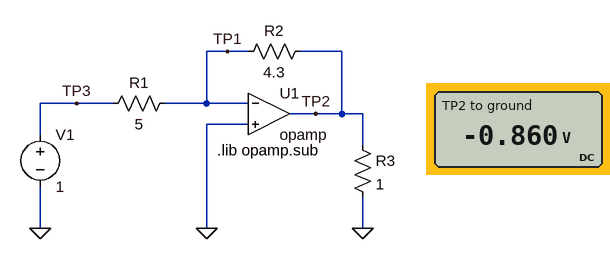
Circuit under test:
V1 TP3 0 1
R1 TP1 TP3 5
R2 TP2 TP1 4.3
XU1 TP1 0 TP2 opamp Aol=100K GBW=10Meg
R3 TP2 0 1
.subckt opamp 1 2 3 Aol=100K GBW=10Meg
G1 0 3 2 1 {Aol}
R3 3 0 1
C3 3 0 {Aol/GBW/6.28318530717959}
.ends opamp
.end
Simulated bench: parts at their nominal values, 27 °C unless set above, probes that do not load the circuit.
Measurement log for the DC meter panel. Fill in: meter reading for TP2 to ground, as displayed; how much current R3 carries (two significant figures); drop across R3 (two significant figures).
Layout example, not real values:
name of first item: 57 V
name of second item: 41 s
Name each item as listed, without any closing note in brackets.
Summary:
meter reading for TP2 to ground, as displayed: -0.860 V
how much current R3 carries: 860 mA
drop across R3: 860 mV
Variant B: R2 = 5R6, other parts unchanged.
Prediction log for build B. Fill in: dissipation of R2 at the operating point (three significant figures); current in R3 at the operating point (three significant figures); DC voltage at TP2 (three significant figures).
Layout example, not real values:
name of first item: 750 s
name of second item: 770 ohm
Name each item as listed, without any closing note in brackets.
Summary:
dissipation of R2 at the operating point: 224 mW
current in R3 at the operating point: 1.12 A
DC voltage at TP2: -1.12 V
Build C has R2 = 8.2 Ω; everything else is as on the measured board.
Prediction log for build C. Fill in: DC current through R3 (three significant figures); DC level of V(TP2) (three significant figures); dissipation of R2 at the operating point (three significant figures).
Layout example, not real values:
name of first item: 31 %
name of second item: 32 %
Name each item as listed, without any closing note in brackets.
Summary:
DC current through R3: 1.64 A
DC level of V(TP2): -1.64 V
dissipation of R2 at the operating point: 328 mW
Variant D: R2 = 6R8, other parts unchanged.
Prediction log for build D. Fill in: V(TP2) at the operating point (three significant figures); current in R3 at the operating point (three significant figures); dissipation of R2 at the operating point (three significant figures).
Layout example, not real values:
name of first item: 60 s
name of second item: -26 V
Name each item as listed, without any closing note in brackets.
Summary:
V(TP2) at the operating point: -1.36 V
current in R3 at the operating point: 1.36 A
dissipation of R2 at the operating point: 272 mW
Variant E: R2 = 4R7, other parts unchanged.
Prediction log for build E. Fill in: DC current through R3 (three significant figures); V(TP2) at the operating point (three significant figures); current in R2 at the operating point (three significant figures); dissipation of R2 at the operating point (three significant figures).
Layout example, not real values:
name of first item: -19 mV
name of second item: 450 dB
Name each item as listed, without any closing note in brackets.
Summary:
DC current through R3: 940 mA
V(TP2) at the operating point: -940 mV
current in R2 at the operating point: 200 mA
dissipation of R2 at the operating point: 188 mW
